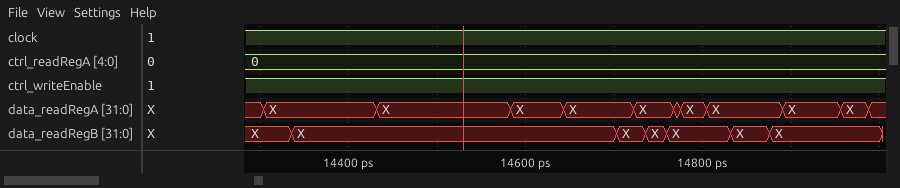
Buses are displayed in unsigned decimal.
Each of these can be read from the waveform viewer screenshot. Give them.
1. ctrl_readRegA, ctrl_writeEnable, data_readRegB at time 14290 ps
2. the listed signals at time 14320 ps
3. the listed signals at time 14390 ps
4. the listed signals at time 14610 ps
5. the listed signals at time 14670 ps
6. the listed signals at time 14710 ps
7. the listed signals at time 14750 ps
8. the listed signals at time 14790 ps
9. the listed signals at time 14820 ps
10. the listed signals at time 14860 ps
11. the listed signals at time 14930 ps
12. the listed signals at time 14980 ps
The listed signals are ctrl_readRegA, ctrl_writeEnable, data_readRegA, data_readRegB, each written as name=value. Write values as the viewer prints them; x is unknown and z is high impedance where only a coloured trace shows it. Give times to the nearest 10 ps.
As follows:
ctrl_readRegA=0, ctrl_writeEnable=1, data_readRegB=X
ctrl_readRegA=0, ctrl_writeEnable=1, data_readRegA=X, data_readRegB=X
ctrl_readRegA=0, ctrl_writeEnable=1, data_readRegA=X, data_readRegB=X
ctrl_readRegA=0, ctrl_writeEnable=1, data_readRegA=X, data_readRegB=X
ctrl_readRegA=0, ctrl_writeEnable=1, data_readRegA=X, data_readRegB=X
ctrl_readRegA=0, ctrl_writeEnable=1, data_readRegA=X, data_readRegB=X
ctrl_readRegA=0, ctrl_writeEnable=1, data_readRegA=X, data_readRegB=X
ctrl_readRegA=0, ctrl_writeEnable=1, data_readRegA=X, data_readRegB=X
ctrl_readRegA=0, ctrl_writeEnable=1, data_readRegA=X, data_readRegB=X
ctrl_readRegA=0, ctrl_writeEnable=1, data_readRegA=X, data_readRegB=X
ctrl_readRegA=0, ctrl_writeEnable=1, data_readRegA=X, data_readRegB=X
ctrl_readRegA=0, ctrl_writeEnable=1, data_readRegA=X, data_readRegB=X
